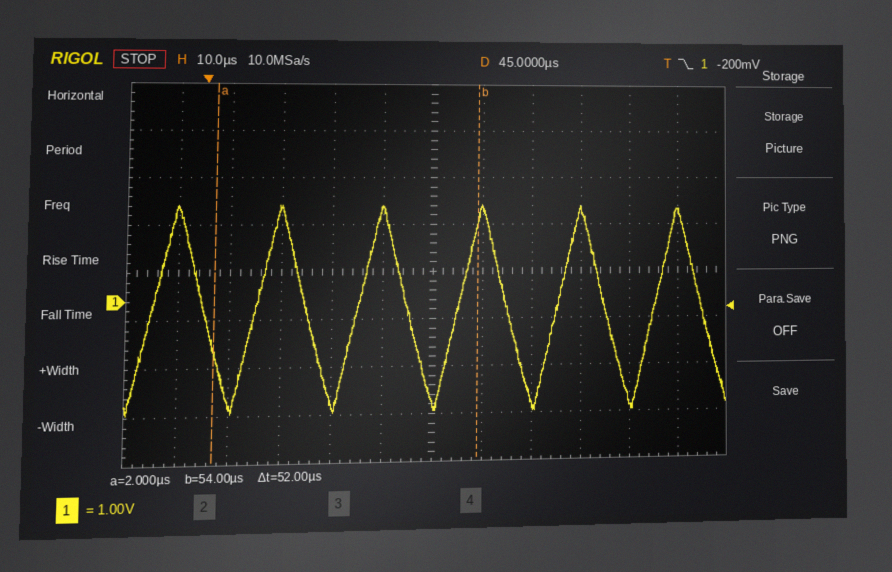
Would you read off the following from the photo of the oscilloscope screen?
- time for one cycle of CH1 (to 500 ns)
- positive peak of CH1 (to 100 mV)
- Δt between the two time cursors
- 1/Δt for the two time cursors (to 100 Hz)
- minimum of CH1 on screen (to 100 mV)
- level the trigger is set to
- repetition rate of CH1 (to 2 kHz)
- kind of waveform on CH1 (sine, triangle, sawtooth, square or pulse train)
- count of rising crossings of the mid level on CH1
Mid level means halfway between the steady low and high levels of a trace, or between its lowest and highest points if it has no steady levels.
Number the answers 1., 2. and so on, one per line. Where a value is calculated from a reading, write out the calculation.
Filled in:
1. 20.0 µs
2. 2.0 V
3. 52 µs
4. 1 / 52 µs ≈ 19.2 kHz
5. -2.3 V
6. -200 mV
7. 1 / 20.0 µs ≈ 50 kHz
8. triangle
9. 6
